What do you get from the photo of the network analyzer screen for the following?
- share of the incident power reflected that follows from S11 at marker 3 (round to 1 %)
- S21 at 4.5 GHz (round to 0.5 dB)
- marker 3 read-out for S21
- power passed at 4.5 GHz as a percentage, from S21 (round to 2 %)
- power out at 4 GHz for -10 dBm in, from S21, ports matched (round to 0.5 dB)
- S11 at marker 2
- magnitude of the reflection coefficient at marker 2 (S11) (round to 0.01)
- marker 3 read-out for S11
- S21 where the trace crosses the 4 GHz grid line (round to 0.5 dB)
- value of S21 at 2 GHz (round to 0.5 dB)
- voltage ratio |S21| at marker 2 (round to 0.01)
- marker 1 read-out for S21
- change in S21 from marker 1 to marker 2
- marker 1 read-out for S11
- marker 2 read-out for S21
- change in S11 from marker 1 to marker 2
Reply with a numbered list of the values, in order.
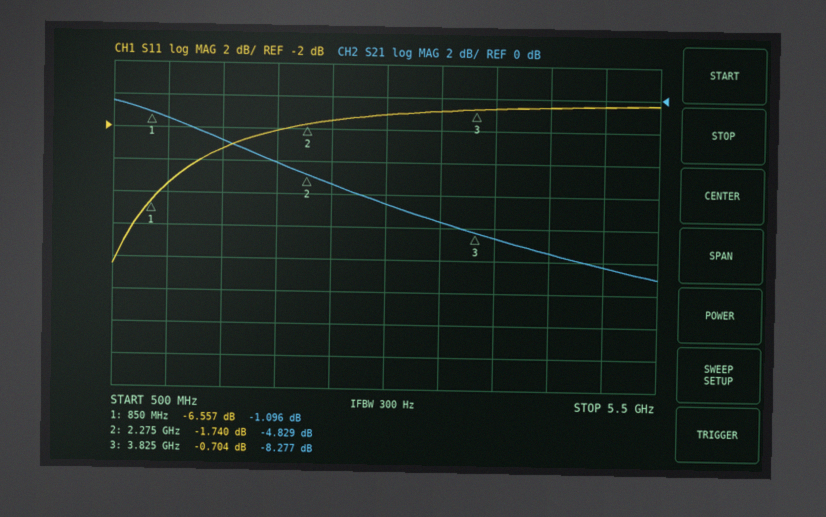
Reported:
1. 85 %
2. -9.5 dB
3. -8.277 dB
4. 12 %
5. -18.5 dBm
6. -1.740 dB
7. 0.82
8. -0.704 dB
9. -8.5 dB
10. -4.0 dB
11. 0.57
12. -1.096 dB
13. -3.733 dB
14. -6.557 dB
15. -4.829 dB
16. 4.817 dB
